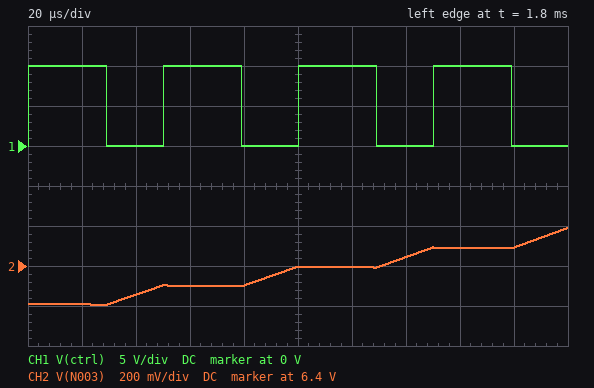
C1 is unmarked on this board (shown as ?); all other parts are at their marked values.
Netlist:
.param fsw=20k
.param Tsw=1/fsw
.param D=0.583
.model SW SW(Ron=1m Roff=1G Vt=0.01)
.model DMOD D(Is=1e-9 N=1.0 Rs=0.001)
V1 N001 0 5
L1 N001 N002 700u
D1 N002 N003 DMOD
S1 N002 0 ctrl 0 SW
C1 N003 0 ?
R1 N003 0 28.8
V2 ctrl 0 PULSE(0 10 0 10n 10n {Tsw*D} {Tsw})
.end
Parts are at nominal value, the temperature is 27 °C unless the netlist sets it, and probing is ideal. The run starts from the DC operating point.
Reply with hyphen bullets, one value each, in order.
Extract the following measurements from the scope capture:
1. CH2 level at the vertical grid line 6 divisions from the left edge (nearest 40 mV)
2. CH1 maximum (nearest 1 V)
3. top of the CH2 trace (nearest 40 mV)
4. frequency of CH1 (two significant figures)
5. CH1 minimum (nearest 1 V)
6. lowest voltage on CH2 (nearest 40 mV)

- 6.40 V
- 10 V
- 6.60 V
- 20 kHz
- 0 V
- 6.20 V
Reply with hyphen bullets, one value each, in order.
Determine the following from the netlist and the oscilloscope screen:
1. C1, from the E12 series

- 1.5 mF
